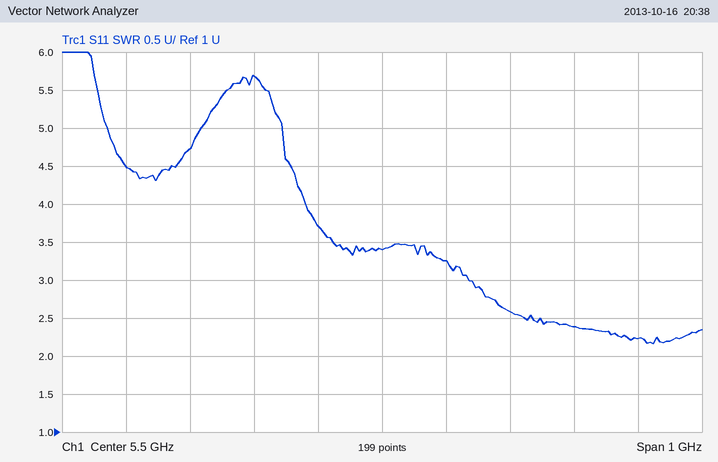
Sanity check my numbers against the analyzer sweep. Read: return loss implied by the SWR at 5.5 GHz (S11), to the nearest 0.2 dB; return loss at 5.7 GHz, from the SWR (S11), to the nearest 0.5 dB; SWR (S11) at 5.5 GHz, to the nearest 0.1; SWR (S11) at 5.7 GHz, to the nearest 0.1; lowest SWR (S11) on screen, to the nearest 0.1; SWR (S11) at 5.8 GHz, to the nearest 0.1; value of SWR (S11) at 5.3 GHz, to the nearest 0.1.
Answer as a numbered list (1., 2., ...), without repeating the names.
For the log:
1. 5.2 dB
2. 7.0 dB
3. 3.4
4. 2.6
5. 2.2
6. 2.4
7. 5.7
